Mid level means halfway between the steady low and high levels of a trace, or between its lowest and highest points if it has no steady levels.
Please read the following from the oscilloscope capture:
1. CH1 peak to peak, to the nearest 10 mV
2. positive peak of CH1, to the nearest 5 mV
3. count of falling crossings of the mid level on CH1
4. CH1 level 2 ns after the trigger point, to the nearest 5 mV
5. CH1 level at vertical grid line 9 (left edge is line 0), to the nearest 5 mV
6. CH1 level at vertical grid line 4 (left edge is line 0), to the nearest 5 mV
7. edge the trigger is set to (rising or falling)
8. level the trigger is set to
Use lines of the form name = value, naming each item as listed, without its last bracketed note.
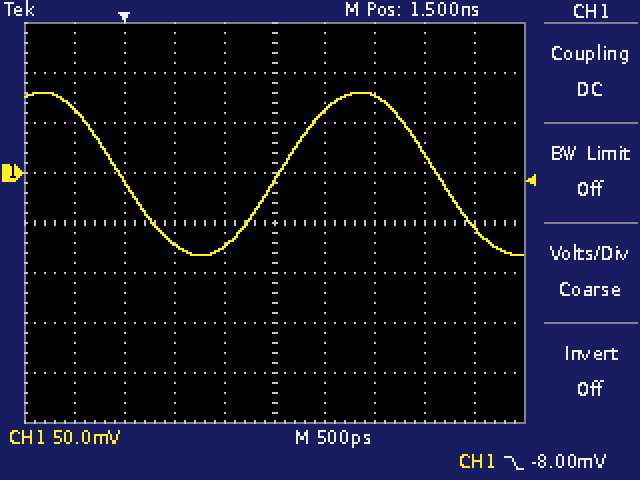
CH1 peak to peak, to the nearest 10 mV = 160 mV
positive peak of CH1, to the nearest 5 mV = 80 mV
count of falling crossings of the mid level on CH1 = 2
CH1 level 2 ns after the trigger point, to the nearest 5 mV = 60 mV
CH1 level at vertical grid line 9 (left edge is line 0), to the nearest 5 mV = -55 mV
CH1 level at vertical grid line 4 (left edge is line 0), to the nearest 5 mV = -75 mV
edge the trigger is set to = falling
level the trigger is set to = -8.00 mV
